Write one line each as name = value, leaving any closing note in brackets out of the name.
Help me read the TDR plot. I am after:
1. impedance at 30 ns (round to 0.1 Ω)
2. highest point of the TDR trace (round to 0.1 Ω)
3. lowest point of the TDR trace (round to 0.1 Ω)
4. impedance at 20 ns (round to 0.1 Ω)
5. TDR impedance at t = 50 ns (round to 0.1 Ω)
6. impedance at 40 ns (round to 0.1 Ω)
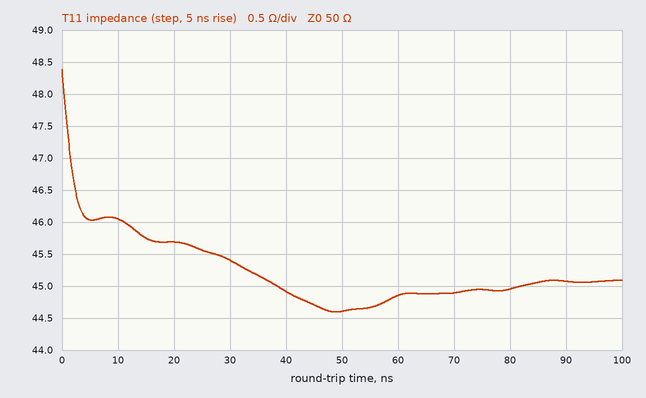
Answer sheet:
impedance at 30 ns = 45.4 Ω
highest point of the TDR trace = 48.4 Ω
lowest point of the TDR trace = 44.6 Ω
impedance at 20 ns = 45.7 Ω
TDR impedance at t = 50 ns = 44.6 Ω
impedance at 40 ns = 44.9 Ω
